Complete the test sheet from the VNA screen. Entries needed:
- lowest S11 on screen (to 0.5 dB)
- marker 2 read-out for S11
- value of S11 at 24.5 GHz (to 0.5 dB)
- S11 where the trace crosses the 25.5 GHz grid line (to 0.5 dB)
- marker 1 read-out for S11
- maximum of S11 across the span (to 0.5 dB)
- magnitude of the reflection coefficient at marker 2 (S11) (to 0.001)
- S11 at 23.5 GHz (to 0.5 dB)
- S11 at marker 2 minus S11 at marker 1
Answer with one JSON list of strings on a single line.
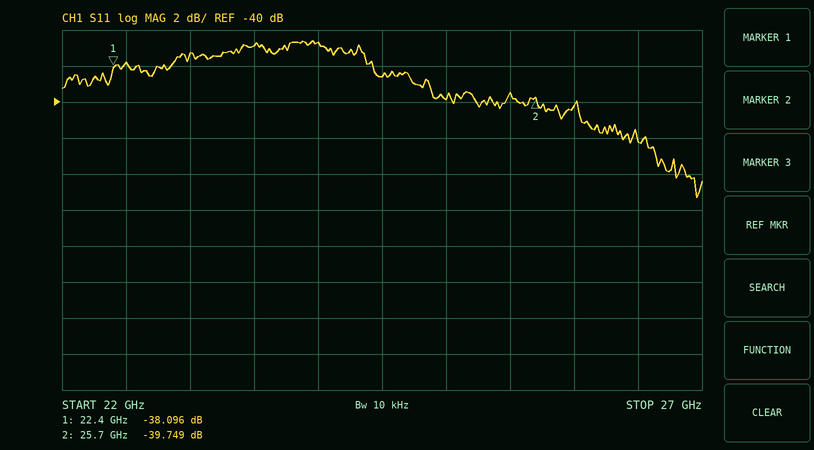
["-45.5 dB", "-39.749 dB", "-38.5 dB", "-39.5 dB", "-38.096 dB", "-36.5 dB", "0.010", "-37.0 dB", "-1.653 dB"]
